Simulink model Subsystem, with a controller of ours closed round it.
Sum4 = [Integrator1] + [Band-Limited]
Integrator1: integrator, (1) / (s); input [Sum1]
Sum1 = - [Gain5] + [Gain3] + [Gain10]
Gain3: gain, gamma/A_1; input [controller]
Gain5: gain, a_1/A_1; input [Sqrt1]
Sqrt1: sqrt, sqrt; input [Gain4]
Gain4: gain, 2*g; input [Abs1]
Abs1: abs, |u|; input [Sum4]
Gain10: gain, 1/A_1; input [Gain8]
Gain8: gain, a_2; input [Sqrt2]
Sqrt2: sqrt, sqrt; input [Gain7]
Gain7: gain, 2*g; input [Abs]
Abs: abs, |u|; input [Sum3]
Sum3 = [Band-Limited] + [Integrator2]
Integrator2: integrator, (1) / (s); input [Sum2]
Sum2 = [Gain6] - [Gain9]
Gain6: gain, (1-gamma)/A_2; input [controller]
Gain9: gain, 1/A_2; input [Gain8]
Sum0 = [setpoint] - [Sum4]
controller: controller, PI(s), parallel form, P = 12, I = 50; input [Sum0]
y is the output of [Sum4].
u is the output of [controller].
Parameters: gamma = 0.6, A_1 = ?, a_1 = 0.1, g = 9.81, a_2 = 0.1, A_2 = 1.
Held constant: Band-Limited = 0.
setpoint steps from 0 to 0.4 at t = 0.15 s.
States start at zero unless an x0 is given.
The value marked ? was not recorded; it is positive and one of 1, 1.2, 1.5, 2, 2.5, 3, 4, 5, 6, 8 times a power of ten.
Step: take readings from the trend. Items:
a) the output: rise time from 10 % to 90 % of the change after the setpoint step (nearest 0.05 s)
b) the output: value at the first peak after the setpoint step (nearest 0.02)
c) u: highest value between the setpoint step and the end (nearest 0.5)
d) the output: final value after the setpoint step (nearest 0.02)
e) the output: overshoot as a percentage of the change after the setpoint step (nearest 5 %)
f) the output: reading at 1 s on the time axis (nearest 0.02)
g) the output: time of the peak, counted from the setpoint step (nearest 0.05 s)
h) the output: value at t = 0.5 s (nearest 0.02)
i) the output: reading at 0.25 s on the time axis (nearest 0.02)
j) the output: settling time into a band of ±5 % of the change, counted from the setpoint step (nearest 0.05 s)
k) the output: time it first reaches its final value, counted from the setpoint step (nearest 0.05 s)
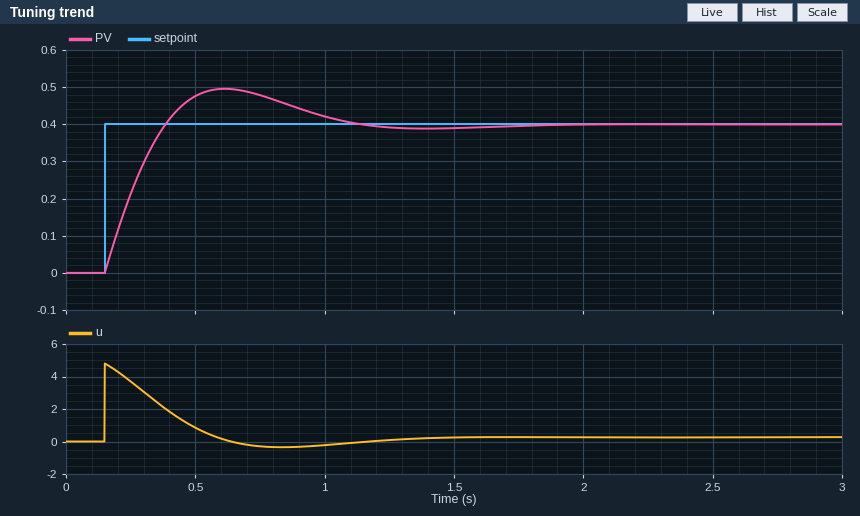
0.20 s
0.50
5.0
0.40
25 %
0.42
0.45 s
0.48
0.22
0.85 s
0.25 s
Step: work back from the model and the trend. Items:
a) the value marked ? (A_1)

1.2
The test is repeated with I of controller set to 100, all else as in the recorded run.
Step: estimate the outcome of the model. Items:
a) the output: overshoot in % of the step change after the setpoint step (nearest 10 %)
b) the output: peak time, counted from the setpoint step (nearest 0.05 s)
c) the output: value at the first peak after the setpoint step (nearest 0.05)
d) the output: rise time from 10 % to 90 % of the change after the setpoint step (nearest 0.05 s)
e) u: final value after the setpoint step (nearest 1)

30 %
0.35 s
0.55
0.15 s
0
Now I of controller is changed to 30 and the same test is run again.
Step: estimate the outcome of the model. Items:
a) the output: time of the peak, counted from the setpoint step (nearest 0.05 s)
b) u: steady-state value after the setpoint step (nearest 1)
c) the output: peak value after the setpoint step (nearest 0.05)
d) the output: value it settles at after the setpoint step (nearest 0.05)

0.55 s
0
0.45
0.40
